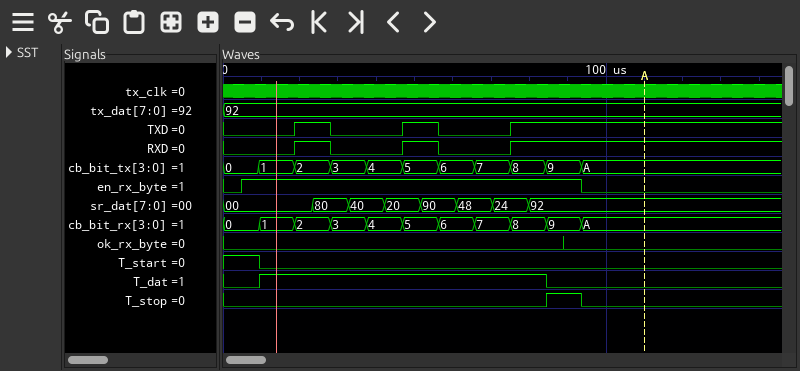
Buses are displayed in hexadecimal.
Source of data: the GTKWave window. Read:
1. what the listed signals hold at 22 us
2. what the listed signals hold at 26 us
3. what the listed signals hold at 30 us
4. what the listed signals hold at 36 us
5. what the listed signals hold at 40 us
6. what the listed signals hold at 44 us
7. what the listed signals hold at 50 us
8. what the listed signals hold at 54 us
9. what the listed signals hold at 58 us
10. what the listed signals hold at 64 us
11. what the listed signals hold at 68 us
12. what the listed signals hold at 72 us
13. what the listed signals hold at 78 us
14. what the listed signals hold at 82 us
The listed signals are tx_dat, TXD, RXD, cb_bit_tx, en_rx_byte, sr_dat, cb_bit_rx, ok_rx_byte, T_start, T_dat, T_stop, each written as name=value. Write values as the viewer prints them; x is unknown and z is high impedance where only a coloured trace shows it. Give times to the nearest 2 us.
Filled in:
tx_dat=92, TXD=1, RXD=1, cb_bit_tx=2, en_rx_byte=1, sr_dat=00, cb_bit_rx=2, ok_rx_byte=0, T_start=0, T_dat=1, T_stop=0
tx_dat=92, TXD=1, RXD=1, cb_bit_tx=2, en_rx_byte=1, sr_dat=80, cb_bit_rx=2, ok_rx_byte=0, T_start=0, T_dat=1, T_stop=0
tx_dat=92, TXD=0, RXD=0, cb_bit_tx=3, en_rx_byte=1, sr_dat=80, cb_bit_rx=3, ok_rx_byte=0, T_start=0, T_dat=1, T_stop=0
tx_dat=92, TXD=0, RXD=0, cb_bit_tx=3, en_rx_byte=1, sr_dat=40, cb_bit_rx=3, ok_rx_byte=0, T_start=0, T_dat=1, T_stop=0
tx_dat=92, TXD=0, RXD=0, cb_bit_tx=4, en_rx_byte=1, sr_dat=40, cb_bit_rx=4, ok_rx_byte=0, T_start=0, T_dat=1, T_stop=0
tx_dat=92, TXD=0, RXD=0, cb_bit_tx=4, en_rx_byte=1, sr_dat=20, cb_bit_rx=4, ok_rx_byte=0, T_start=0, T_dat=1, T_stop=0
tx_dat=92, TXD=1, RXD=1, cb_bit_tx=5, en_rx_byte=1, sr_dat=20, cb_bit_rx=5, ok_rx_byte=0, T_start=0, T_dat=1, T_stop=0
tx_dat=92, TXD=1, RXD=1, cb_bit_tx=5, en_rx_byte=1, sr_dat=90, cb_bit_rx=5, ok_rx_byte=0, T_start=0, T_dat=1, T_stop=0
tx_dat=92, TXD=0, RXD=0, cb_bit_tx=6, en_rx_byte=1, sr_dat=90, cb_bit_rx=6, ok_rx_byte=0, T_start=0, T_dat=1, T_stop=0
tx_dat=92, TXD=0, RXD=0, cb_bit_tx=6, en_rx_byte=1, sr_dat=48, cb_bit_rx=6, ok_rx_byte=0, T_start=0, T_dat=1, T_stop=0
tx_dat=92, TXD=0, RXD=0, cb_bit_tx=7, en_rx_byte=1, sr_dat=48, cb_bit_rx=7, ok_rx_byte=0, T_start=0, T_dat=1, T_stop=0
tx_dat=92, TXD=0, RXD=0, cb_bit_tx=7, en_rx_byte=1, sr_dat=24, cb_bit_rx=7, ok_rx_byte=0, T_start=0, T_dat=1, T_stop=0
tx_dat=92, TXD=1, RXD=1, cb_bit_tx=8, en_rx_byte=1, sr_dat=24, cb_bit_rx=8, ok_rx_byte=0, T_start=0, T_dat=1, T_stop=0
tx_dat=92, TXD=1, RXD=1, cb_bit_tx=8, en_rx_byte=1, sr_dat=92, cb_bit_rx=8, ok_rx_byte=0, T_start=0, T_dat=1, T_stop=0
